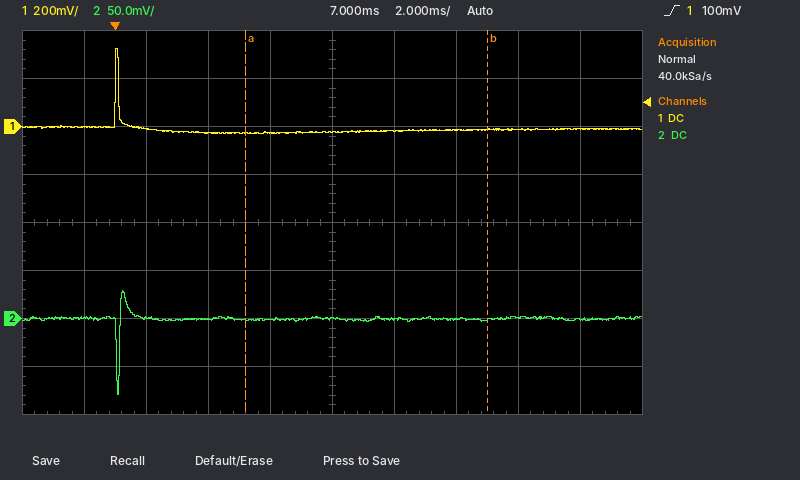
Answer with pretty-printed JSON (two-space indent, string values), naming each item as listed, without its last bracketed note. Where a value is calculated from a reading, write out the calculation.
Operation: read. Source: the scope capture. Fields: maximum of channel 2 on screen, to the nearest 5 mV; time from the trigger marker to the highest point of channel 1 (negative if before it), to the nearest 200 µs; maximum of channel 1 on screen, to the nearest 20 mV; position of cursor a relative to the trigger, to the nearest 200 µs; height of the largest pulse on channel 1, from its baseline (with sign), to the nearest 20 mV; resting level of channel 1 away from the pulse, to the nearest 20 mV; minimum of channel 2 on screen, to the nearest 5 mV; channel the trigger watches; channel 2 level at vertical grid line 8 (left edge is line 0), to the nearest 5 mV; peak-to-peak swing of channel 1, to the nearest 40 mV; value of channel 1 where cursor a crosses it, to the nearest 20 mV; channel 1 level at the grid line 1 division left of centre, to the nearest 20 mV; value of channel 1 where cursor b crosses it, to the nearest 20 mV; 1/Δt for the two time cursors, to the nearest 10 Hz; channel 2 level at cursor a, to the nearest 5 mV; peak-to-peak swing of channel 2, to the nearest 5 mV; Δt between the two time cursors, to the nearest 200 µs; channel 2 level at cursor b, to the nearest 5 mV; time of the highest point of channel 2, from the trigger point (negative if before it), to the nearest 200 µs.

{
  "maximum of channel 2 on screen, to the nearest 5 mV": "30 mV",
  "time from the trigger marker to the highest point of channel 1 (negative if before it), to the nearest 200 µs": "0.0 ms",
  "maximum of channel 1 on screen, to the nearest 20 mV": "320 mV",
  "position of cursor a relative to the trigger, to the nearest 200 µs": "+4.2 ms",
  "height of the largest pulse on channel 1, from its baseline (with sign), to the nearest 20 mV": "320 mV − (-20 mV) = +340 mV",
  "resting level of channel 1 away from the pulse, to the nearest 20 mV": "-20 mV",
  "minimum of channel 2 on screen, to the nearest 5 mV": "-80 mV",
  "channel the trigger watches": "channel 1",
  "channel 2 level at vertical grid line 8 (left edge is line 0), to the nearest 5 mV": "0 mV",
  "peak-to-peak swing of channel 1, to the nearest 40 mV": "360 mV",
  "value of channel 1 where cursor a crosses it, to the nearest 20 mV": "-20 mV",
  "channel 1 level at the grid line 1 division left of centre, to the nearest 20 mV": "-20 mV",
  "value of channel 1 where cursor b crosses it, to the nearest 20 mV": "-20 mV",
  "1/Δt for the two time cursors, to the nearest 10 Hz": "1 / 7.8 ms ≈ 130 Hz",
  "channel 2 level at cursor a, to the nearest 5 mV": "0 mV",
  "peak-to-peak swing of channel 2, to the nearest 5 mV": "30 mV − (-80 mV) = 110 mV",
  "Δt between the two time cursors, to the nearest 200 µs": "7.8 ms",
  "channel 2 level at cursor b, to the nearest 5 mV": "0 mV",
  "time of the highest point of channel 2, from the trigger point (negative if before it), to the nearest 200 µs": "+200 µs"
}
